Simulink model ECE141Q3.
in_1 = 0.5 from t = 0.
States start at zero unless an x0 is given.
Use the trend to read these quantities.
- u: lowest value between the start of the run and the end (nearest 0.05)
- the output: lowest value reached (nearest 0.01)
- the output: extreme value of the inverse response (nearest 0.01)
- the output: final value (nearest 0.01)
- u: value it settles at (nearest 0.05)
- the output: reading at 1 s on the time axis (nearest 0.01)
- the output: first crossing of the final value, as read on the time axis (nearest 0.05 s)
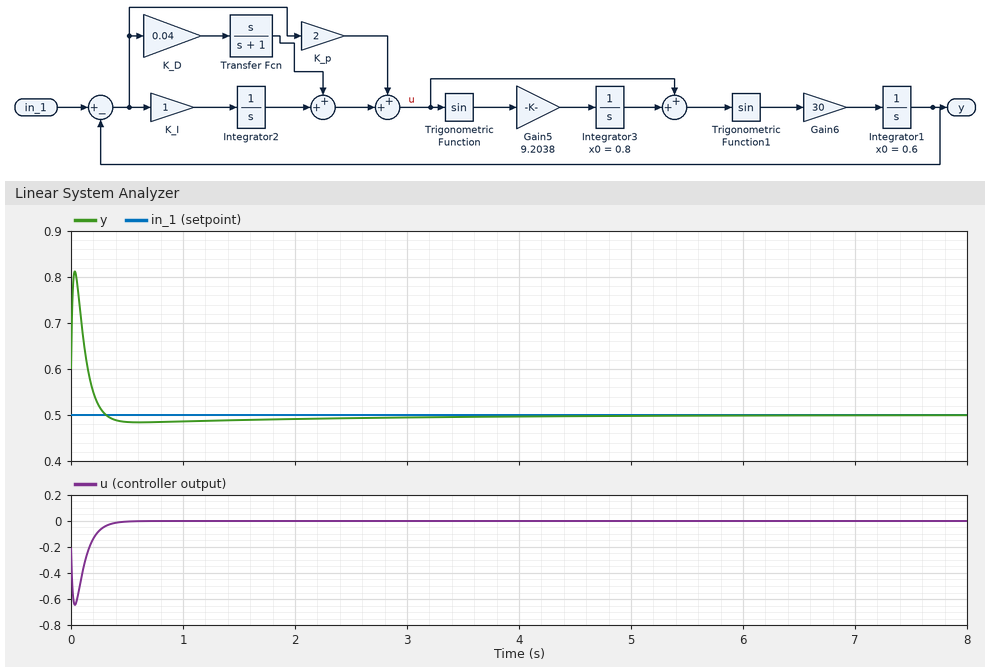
-0.65
0.48
0.81
0.50
0.00
0.49
0.30 s
